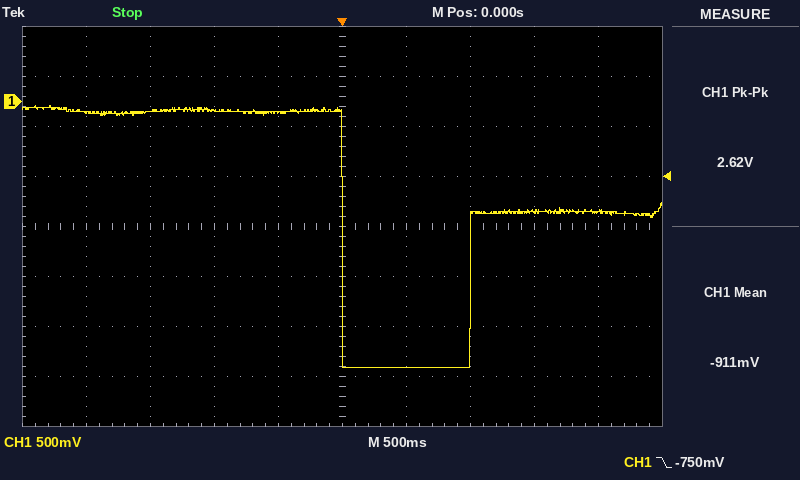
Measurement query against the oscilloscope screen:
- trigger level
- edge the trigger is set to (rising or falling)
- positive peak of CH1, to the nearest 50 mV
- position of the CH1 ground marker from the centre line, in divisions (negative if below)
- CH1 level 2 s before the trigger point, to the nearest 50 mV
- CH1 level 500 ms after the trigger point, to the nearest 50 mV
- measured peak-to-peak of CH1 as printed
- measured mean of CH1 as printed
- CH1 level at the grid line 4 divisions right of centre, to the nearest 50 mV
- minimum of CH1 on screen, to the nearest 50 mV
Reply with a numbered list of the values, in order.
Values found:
1. -750 mV
2. falling
3. -50 mV
4. +2.5 div
5. -100 mV
6. -2.65 V
7. 2.62 V
8. -911 mV
9. -1.10 V
10. -2.65 V
